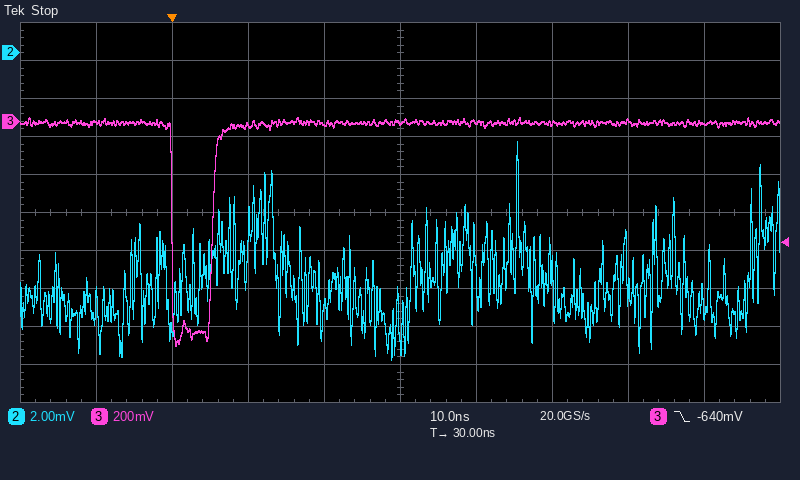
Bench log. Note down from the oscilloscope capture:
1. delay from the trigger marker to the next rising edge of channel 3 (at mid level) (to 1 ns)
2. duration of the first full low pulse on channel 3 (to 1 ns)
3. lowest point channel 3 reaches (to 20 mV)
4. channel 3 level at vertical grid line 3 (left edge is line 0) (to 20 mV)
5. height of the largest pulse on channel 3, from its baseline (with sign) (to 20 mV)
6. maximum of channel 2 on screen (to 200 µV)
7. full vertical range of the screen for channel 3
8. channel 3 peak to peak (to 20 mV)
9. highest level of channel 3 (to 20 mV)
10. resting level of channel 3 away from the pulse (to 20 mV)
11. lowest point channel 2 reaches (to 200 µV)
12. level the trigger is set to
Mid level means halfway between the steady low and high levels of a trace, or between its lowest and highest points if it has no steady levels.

5 ns
5 ns
-1.18 V
-20 mV
-1.18 V
-4.6 mV
2 V
1.20 V
20 mV
0 mV
-16.2 mV
-640 mV
